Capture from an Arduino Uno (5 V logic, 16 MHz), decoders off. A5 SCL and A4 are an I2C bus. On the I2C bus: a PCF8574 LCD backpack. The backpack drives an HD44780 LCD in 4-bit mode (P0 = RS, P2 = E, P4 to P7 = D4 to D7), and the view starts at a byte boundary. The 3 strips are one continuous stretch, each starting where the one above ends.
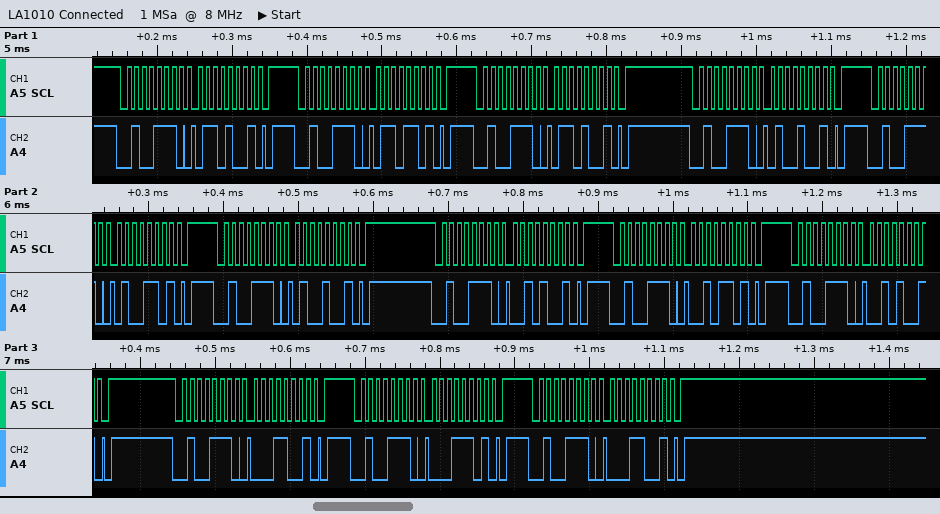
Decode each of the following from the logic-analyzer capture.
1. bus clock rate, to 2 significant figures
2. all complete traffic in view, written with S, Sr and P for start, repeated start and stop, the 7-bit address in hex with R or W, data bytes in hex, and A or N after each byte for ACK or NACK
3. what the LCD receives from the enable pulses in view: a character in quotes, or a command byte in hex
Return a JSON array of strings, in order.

["100 kHz", "S 27W A 69 A P S 27W A 6D A P S 27W A 69 A P S 27W A 49 A P S 27W A 4D A P S 27W A 49 A P S 27W A 29 A P S 27W A 2D A P S 27W A 29 A P S 27W A 19 A P S 27W A 1D A P S 27W A 19 A P", "'d' '!'"]
